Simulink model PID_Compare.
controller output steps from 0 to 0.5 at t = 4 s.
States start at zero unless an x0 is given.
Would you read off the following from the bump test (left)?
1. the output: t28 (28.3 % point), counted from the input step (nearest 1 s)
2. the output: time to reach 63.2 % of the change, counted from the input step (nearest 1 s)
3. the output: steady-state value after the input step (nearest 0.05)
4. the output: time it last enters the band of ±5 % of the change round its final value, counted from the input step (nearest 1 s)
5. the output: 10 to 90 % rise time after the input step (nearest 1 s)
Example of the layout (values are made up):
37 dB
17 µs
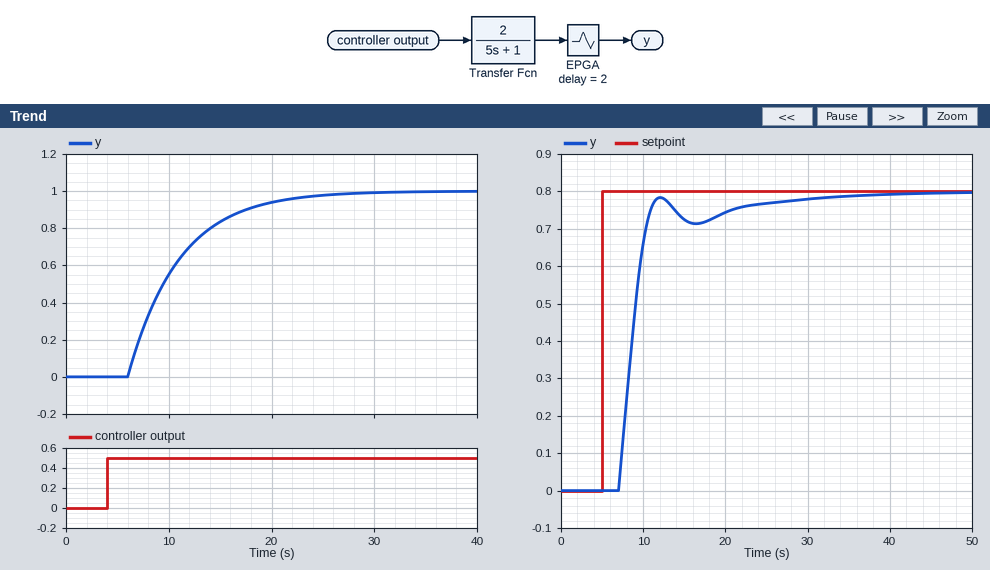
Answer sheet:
4 s
7 s
1.00
17 s
11 s
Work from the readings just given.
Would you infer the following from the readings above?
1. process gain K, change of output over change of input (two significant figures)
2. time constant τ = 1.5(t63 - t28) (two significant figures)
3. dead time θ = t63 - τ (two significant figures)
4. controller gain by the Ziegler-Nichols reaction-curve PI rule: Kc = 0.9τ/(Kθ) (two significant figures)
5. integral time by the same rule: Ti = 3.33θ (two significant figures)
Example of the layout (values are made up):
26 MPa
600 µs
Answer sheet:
2.0
4.5 s
2.5 s
0.81
8.3 s
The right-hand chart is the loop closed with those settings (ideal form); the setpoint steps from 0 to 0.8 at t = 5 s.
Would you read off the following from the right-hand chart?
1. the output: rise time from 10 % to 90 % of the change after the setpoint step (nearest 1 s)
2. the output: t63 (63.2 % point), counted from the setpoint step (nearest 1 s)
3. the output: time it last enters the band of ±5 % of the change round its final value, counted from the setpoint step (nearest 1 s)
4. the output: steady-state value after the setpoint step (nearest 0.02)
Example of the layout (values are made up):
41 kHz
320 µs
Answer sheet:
3 s
4 s
17 s
0.80
